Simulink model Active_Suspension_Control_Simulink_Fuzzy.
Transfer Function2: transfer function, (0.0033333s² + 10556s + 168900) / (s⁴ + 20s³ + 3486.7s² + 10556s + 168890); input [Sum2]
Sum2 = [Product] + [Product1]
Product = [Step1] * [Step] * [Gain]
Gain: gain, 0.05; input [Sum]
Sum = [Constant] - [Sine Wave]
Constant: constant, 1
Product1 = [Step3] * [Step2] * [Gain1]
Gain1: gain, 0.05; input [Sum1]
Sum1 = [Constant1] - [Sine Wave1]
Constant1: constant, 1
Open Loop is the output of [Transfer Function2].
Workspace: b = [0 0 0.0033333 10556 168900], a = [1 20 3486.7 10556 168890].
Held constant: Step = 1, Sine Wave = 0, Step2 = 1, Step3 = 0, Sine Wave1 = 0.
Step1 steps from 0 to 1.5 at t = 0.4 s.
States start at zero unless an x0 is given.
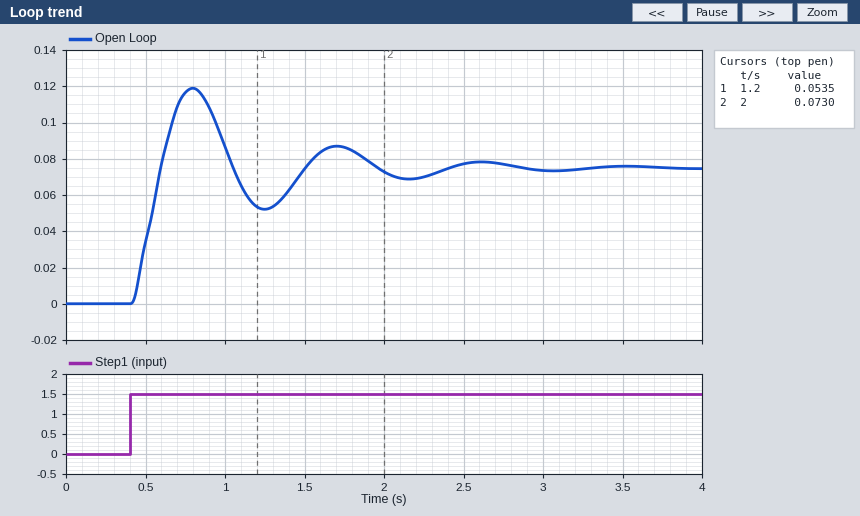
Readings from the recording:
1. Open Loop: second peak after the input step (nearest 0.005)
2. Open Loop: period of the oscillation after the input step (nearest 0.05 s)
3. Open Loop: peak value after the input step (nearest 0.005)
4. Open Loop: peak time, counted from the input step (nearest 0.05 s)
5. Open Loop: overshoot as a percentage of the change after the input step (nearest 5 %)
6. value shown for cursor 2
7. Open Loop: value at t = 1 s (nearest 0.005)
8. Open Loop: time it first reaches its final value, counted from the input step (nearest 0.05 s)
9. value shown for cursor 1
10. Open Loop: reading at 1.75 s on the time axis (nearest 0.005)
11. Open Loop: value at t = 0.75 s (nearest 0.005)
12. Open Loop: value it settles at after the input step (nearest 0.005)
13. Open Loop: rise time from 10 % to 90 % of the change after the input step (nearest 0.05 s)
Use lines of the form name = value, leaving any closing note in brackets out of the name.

Open Loop: second peak after the input step = 0.085
Open Loop: period of the oscillation after the input step = 0.90 s
Open Loop: peak value after the input step = 0.120
Open Loop: peak time, counted from the input step = 0.40 s
Open Loop: overshoot as a percentage of the change after the input step = 60 %
value shown for cursor 2 = 0.0730
Open Loop: value at t = 1 s = 0.085
Open Loop: time it first reaches its final value, counted from the input step = 0.20 s
value shown for cursor 1 = 0.0535
Open Loop: reading at 1.75 s on the time axis = 0.085
Open Loop: value at t = 0.75 s = 0.115
Open Loop: value it settles at after the input step = 0.075
Open Loop: rise time from 10 % to 90 % of the change after the input step = 0.15 s
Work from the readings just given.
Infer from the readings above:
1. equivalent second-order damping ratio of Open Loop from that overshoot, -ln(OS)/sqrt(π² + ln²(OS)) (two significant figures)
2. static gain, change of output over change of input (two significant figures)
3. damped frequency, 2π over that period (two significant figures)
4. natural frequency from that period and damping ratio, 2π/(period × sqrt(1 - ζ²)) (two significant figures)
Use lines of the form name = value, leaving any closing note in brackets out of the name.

equivalent second-order damping ratio of Open Loop from that overshoot, -ln(OS)/sqrt(π² + ln²(OS)) = 0.16
static gain, change of output over change of input = 0.050
damped frequency, 2π over that period = 7.0 rad/s
natural frequency from that period and damping ratio, 2π/(period × sqrt(1 - ζ²)) = 7.1 rad/s
